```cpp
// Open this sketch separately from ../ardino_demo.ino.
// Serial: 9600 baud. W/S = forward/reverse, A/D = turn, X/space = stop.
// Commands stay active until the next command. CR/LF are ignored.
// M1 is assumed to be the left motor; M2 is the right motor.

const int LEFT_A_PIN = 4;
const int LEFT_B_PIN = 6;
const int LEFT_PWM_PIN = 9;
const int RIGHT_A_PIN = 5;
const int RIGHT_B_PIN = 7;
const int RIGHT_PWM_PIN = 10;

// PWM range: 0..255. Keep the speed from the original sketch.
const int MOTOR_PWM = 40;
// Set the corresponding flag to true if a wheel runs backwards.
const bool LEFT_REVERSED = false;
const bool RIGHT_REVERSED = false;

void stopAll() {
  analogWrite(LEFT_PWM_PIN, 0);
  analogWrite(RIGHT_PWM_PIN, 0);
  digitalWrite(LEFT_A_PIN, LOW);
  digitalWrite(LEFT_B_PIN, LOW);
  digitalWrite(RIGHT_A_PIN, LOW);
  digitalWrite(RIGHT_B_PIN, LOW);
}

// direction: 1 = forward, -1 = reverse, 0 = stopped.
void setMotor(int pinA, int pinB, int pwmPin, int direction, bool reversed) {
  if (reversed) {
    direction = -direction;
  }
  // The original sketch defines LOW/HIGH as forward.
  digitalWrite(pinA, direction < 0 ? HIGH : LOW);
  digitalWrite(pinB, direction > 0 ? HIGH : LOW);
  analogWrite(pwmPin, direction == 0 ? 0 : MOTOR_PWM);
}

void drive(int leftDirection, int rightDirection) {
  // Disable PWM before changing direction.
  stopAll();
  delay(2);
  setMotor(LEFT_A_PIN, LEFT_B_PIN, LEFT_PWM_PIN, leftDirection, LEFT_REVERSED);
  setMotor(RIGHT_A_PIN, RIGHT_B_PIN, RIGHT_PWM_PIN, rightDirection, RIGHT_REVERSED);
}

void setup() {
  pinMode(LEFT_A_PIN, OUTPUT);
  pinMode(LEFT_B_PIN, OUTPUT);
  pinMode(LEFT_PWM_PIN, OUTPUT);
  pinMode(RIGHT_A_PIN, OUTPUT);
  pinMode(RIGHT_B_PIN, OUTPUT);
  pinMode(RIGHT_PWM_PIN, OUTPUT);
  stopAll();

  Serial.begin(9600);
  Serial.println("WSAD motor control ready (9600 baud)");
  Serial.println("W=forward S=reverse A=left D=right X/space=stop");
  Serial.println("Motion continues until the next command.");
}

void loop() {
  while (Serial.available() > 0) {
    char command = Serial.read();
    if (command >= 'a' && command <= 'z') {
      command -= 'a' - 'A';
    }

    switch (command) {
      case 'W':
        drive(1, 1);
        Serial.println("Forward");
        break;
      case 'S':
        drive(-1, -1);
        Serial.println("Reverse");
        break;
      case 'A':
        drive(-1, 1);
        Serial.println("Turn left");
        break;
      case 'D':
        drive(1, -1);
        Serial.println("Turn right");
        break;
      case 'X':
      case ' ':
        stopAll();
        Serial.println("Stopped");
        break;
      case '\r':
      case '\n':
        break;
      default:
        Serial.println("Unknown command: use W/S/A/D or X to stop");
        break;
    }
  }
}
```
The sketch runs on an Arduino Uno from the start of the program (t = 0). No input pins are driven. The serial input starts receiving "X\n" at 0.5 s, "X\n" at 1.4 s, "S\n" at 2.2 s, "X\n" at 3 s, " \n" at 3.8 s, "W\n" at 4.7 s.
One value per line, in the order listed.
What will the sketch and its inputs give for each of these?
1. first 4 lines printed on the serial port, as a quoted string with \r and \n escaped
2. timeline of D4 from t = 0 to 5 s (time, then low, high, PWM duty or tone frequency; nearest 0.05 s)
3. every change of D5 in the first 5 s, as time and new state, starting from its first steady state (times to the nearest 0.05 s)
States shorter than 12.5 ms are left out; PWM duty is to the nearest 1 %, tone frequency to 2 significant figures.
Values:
"WSAD motor control ready (9600 baud)\r\nW=forward S=reverse A=left D=right X/space=stop\r\nMotion continues until the next command.\r\nStopped\r\n"
0 s low; 2.2 s high; 3 s low
0 s low; 2.2 s high; 3 s low
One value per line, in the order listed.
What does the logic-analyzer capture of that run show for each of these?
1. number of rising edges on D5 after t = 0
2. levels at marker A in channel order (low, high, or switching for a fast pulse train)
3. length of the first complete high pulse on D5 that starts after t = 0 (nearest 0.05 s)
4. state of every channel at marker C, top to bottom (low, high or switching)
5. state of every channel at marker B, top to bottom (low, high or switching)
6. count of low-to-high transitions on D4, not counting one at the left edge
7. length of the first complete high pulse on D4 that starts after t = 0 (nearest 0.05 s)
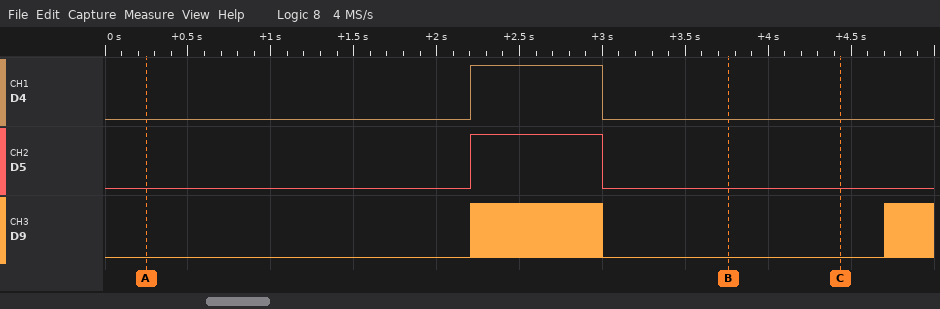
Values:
1
D4 low, D5 low, D9 low
0.80 s
D4 low, D5 low, D9 low
D4 low, D5 low, D9 low
1
0.80 s
